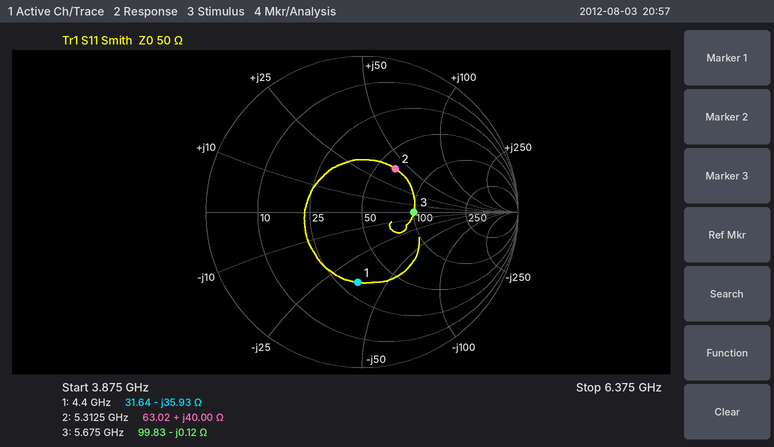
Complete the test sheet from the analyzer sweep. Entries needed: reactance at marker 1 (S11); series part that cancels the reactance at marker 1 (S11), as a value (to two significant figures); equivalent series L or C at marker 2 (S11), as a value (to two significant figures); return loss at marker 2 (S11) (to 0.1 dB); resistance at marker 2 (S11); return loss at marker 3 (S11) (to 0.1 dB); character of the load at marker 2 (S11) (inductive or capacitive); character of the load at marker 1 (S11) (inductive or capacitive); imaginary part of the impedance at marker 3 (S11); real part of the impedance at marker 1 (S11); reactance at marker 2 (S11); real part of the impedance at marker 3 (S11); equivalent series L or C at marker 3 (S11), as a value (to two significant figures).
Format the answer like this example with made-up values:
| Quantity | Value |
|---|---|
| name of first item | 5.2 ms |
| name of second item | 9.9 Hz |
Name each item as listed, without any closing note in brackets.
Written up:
| Quantity | Value |
|---|---|
| reactance at marker 1 | -35.93 Ω |
| series part that cancels the reactance at marker 1 (S11), as a value | 1.3 nH |
| equivalent series L or C at marker 2 (S11), as a value | 1.2 nH |
| return loss at marker 2 (S11) | 9.1 dB |
| resistance at marker 2 | 63.02 Ω |
| return loss at marker 3 (S11) | 9.6 dB |
| character of the load at marker 2 (S11) | inductive |
| character of the load at marker 1 (S11) | capacitive |
| imaginary part of the impedance at marker 3 | -0.12 Ω |
| real part of the impedance at marker 1 | 31.64 Ω |
| reactance at marker 2 | +40.00 Ω |
| real part of the impedance at marker 3 | 99.83 Ω |
| equivalent series L or C at marker 3 (S11), as a value | 230 pF |
